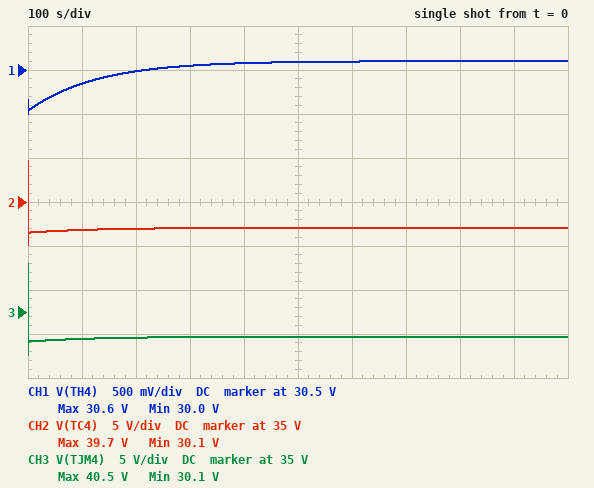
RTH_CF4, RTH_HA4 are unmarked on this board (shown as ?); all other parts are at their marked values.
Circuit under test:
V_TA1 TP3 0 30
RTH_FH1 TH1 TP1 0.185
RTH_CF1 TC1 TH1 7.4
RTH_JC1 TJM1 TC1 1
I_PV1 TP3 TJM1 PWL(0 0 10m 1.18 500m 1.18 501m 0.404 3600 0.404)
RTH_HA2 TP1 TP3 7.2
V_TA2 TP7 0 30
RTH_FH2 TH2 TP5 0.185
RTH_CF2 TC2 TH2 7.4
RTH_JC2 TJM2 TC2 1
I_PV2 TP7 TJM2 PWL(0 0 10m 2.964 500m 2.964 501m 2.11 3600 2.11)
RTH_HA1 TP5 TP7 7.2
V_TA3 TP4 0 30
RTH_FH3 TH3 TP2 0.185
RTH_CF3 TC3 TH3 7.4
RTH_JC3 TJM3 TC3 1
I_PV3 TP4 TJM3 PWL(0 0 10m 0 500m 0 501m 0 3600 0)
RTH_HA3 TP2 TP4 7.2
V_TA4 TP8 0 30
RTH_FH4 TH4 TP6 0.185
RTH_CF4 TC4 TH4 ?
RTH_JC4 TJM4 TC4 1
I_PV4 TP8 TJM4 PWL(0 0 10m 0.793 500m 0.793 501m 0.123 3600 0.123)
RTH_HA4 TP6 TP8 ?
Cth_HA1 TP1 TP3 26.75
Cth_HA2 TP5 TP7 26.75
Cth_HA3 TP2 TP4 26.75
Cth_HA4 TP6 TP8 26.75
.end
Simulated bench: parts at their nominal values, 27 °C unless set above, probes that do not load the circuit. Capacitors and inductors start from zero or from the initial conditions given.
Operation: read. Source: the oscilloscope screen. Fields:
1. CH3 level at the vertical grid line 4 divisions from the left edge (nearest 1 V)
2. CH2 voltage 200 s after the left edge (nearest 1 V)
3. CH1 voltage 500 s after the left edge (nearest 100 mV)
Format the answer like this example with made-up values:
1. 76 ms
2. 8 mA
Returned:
1. 32 V
2. 32 V
3. 30.6 V
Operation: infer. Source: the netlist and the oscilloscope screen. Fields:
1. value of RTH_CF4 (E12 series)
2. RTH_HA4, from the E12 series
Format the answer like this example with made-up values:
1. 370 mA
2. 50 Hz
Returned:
1. 12 Ω
2. 4.7 Ω
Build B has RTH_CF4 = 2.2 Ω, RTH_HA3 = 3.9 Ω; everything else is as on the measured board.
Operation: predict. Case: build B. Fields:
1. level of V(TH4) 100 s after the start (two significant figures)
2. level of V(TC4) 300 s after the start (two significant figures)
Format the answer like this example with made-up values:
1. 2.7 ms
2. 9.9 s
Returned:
1. 30 V
2. 31 V
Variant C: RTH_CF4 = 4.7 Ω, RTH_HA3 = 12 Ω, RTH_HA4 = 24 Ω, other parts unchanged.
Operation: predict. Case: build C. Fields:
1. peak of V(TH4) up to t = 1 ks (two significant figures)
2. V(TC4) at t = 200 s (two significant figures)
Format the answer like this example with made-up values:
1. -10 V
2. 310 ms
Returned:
1. 32 V
2. 31 V
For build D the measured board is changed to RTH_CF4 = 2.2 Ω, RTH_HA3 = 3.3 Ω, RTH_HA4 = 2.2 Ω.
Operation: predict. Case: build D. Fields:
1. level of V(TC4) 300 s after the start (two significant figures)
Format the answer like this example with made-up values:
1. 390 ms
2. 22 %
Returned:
1. 31 V
